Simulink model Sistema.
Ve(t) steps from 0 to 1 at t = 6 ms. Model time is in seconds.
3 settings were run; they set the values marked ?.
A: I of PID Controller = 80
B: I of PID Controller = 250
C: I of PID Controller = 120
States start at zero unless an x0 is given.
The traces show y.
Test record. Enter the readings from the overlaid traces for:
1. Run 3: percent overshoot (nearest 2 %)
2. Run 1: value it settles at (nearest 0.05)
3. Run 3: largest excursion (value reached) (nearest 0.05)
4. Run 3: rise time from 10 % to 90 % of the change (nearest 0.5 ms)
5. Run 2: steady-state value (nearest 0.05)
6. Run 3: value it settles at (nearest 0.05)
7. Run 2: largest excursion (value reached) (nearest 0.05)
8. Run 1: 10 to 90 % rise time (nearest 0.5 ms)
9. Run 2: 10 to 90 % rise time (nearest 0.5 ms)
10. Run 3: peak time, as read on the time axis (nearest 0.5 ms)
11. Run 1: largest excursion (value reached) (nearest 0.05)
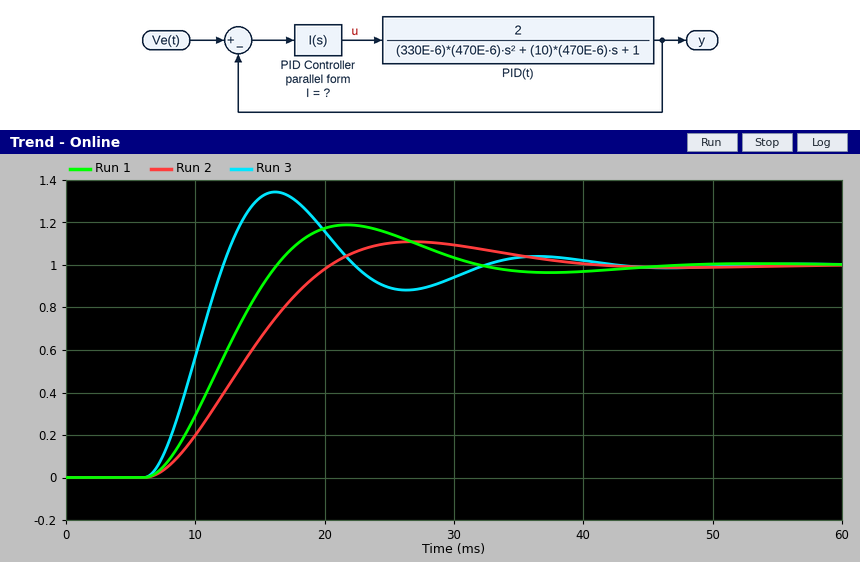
34 %
1.00
1.35
4.0 ms
1.00
1.00
1.10
7.0 ms
9.5 ms
16.0 ms
1.20
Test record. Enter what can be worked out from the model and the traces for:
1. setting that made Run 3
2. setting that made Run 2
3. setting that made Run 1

B
A
C
